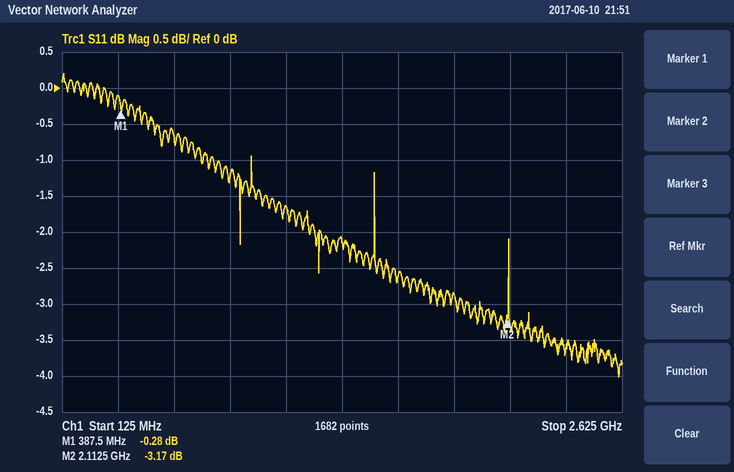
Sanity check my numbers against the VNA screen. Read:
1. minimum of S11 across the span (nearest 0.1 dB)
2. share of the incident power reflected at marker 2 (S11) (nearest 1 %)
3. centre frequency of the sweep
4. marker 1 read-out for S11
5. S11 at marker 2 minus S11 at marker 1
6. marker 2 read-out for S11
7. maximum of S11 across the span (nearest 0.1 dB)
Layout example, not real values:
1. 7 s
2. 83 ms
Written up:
1. -4.0 dB
2. 48 %
3. 1.375 GHz
4. -0.28 dB
5. -2.89 dB
6. -3.17 dB
7. 0.2 dB
